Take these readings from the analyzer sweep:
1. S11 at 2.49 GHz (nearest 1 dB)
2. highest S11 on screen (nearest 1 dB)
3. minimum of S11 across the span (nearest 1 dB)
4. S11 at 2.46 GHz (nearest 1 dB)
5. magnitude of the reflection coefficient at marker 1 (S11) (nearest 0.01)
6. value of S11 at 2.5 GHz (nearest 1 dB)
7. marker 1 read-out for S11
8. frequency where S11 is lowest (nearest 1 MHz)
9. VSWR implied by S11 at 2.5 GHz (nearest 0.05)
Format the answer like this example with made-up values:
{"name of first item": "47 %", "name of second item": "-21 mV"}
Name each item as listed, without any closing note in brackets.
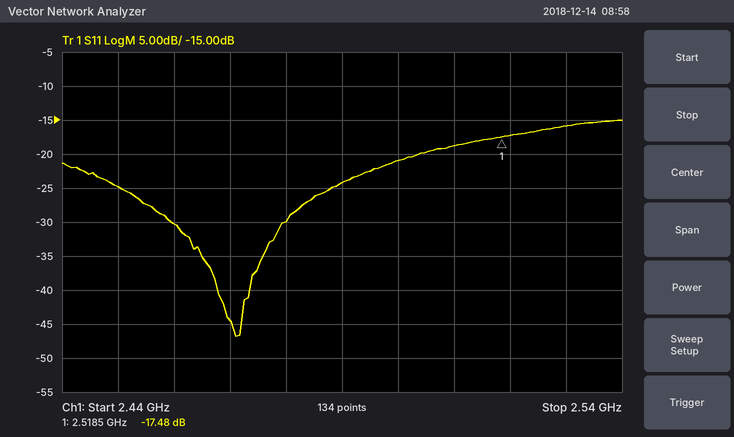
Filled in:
{"S11 at 2.49 GHz": "-24 dB", "highest S11 on screen": "-15 dB", "minimum of S11 across the span": "-47 dB", "S11 at 2.46 GHz": "-30 dB", "magnitude of the reflection coefficient at marker 1 (S11)": "0.13", "value of S11 at 2.5 GHz": "-21 dB", "marker 1 read-out for S11": "-17.48 dB", "frequency where S11 is lowest": "2.471 GHz", "VSWR implied by S11 at 2.5 GHz": "1.20"}
